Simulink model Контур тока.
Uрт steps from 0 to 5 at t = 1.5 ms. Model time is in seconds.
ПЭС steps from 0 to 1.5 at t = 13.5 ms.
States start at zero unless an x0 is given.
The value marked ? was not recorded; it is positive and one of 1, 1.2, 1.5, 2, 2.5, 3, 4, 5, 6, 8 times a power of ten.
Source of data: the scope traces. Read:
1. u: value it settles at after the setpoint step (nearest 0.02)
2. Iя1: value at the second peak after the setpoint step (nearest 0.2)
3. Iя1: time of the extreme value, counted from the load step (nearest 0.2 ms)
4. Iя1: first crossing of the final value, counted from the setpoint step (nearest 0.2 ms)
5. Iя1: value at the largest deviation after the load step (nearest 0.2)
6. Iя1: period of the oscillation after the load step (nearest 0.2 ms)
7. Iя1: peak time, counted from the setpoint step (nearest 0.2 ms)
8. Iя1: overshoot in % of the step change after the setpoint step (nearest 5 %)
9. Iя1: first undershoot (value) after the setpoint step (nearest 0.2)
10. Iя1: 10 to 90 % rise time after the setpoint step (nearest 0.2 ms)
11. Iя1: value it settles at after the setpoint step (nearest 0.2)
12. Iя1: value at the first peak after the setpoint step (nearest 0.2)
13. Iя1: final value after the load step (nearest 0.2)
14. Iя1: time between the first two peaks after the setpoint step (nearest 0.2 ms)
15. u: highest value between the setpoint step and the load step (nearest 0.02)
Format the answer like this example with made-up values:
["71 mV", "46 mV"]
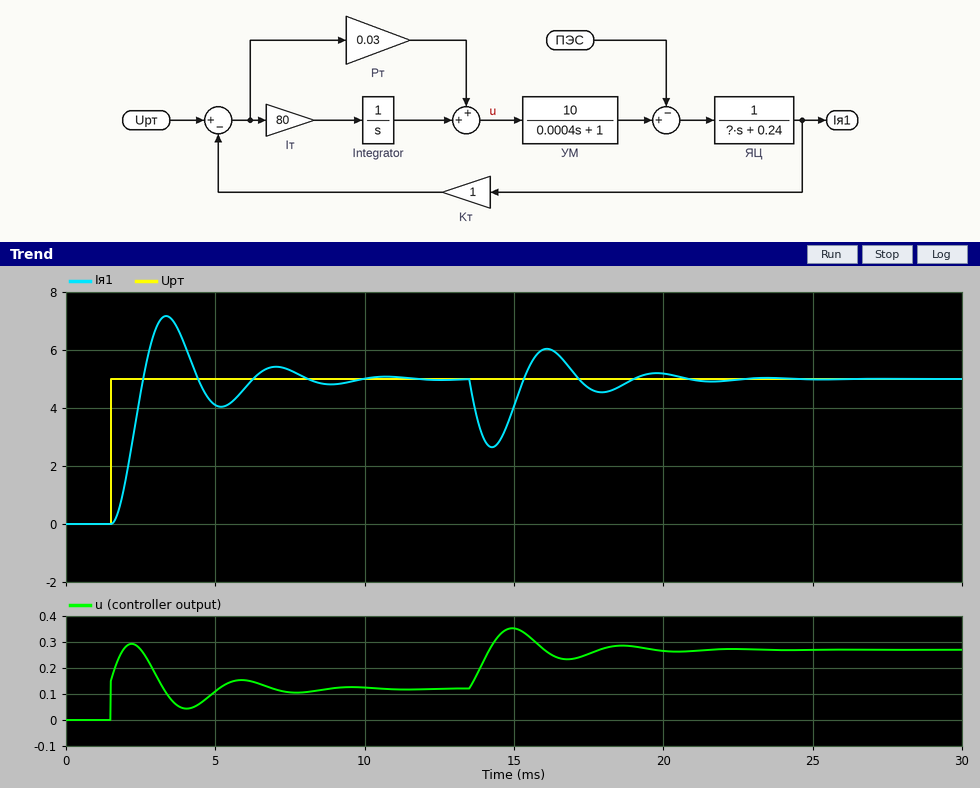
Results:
["0.12", "5.4", "0.8 ms", "1.0 ms", "2.6", "3.6 ms", "1.8 ms", "45 %", "4.0", "0.8 ms", "5.0", "7.2", "5.0", "3.6 ms", "0.30"]
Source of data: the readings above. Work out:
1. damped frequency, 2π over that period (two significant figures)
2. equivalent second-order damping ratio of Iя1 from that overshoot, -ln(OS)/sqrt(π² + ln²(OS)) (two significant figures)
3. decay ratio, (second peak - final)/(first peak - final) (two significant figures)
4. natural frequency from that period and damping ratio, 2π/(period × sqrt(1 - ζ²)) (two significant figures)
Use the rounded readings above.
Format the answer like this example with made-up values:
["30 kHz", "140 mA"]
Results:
["1.7 rad/ms", "0.25", "0.18", "1.8 rad/ms"]
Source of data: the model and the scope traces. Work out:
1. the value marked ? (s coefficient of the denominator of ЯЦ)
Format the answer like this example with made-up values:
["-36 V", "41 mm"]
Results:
["0.00025"]
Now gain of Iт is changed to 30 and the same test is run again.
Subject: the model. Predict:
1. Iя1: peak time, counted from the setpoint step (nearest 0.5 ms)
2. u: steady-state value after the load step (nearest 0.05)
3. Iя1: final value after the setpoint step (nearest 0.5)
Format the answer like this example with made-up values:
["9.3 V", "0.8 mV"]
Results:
["2.5 ms", "0.25", "5.0"]
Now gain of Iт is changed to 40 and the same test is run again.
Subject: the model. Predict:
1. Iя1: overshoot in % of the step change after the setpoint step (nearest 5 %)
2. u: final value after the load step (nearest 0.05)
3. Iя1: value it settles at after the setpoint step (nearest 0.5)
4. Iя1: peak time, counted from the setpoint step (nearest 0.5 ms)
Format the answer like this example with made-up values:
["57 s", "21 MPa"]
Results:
["15 %", "0.25", "5.0", "2.5 ms"]
